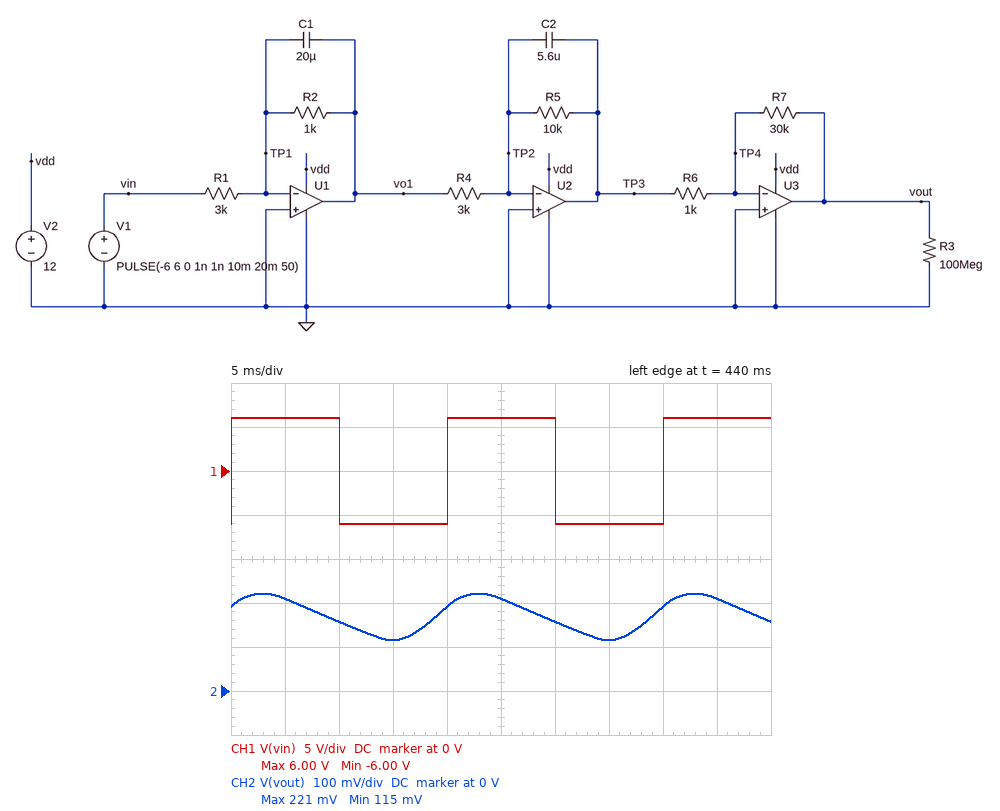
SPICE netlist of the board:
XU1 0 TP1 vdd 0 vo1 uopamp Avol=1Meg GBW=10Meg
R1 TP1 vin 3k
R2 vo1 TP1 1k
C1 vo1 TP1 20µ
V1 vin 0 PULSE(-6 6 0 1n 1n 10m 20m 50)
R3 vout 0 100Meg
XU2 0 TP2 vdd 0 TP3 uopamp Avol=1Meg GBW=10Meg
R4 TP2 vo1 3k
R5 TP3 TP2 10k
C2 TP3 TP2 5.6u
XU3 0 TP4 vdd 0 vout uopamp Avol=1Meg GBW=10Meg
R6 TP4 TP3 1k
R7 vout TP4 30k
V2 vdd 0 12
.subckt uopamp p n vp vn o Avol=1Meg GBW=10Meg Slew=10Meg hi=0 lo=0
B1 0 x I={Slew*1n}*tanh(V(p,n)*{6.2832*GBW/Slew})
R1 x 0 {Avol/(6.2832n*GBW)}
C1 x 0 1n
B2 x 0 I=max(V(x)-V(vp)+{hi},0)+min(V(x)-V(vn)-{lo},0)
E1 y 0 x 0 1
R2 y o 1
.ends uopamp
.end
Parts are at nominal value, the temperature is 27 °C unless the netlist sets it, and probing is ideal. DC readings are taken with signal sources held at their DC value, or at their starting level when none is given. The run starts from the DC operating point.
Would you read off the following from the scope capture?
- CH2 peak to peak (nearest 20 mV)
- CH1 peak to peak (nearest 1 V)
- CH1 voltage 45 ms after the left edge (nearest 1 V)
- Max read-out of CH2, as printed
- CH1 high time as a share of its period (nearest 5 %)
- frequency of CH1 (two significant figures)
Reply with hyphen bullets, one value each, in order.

- 100 mV
- 12 V
- 6 V
- 221 mV
- 50 %
- 50 Hz
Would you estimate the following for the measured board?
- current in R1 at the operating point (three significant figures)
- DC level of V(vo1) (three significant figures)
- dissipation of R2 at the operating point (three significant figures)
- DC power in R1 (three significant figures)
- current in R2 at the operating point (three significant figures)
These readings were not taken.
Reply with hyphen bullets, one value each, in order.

- 2.00 mA
- 2.00 V
- 4.00 mW
- 12.0 mW
- 2.00 mA
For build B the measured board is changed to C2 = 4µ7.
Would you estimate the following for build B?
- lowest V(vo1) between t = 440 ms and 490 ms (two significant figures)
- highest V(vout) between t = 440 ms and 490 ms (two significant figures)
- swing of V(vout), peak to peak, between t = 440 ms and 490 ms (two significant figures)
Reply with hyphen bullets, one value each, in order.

- -12 mV
- 230 mV
- 120 mV
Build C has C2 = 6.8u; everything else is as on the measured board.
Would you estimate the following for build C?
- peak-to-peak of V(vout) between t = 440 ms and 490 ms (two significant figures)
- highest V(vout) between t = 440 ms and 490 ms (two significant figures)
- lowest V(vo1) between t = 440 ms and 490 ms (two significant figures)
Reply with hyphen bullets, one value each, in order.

- 88 mV
- 210 mV
- -12 mV
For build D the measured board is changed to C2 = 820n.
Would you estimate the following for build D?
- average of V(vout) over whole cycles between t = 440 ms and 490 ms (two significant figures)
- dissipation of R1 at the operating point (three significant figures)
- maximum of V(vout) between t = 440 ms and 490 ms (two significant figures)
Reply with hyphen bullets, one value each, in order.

- 130 mV
- 12.0 mW
- 290 mV
